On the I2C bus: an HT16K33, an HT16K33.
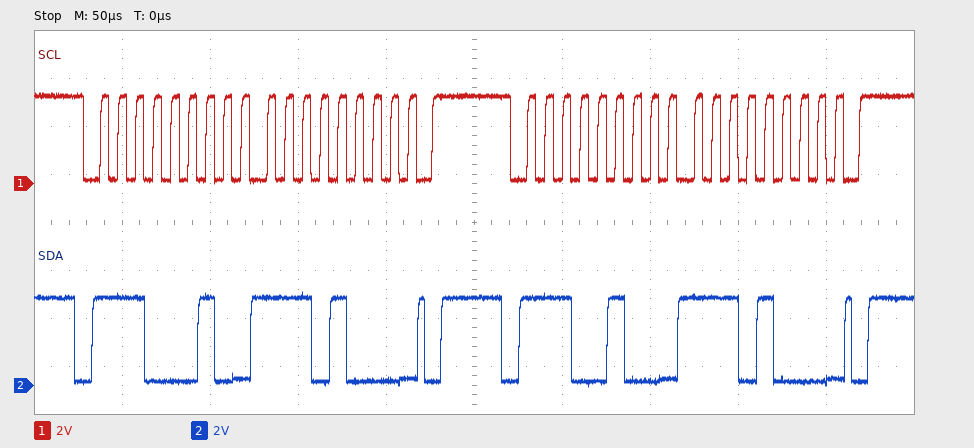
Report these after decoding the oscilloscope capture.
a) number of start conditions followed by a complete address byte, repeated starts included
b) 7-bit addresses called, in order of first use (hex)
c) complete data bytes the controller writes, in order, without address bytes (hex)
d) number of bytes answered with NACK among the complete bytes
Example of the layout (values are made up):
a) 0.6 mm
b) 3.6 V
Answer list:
a) 2
b) 0x71 0x72
c) E8 E8
d) 0
